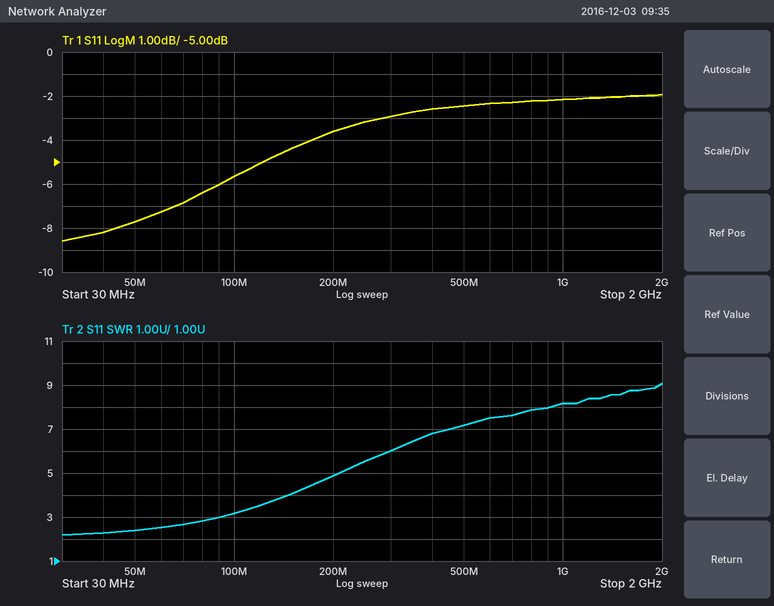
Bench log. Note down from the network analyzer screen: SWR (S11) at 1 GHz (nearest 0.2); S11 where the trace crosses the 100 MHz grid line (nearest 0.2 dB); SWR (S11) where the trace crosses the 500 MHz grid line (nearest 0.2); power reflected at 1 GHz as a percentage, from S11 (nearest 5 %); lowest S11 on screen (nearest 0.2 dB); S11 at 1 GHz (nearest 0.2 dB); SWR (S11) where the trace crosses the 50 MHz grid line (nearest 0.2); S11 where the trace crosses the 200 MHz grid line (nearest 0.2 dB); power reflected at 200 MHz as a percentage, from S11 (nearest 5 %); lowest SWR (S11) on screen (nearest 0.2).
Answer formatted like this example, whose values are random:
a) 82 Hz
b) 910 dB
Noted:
a) 8.2
b) -5.6 dB
c) 7.2
d) 60 %
e) -8.6 dB
f) -2.2 dB
g) 2.4
h) -3.6 dB
i) 45 %
j) 2.2
